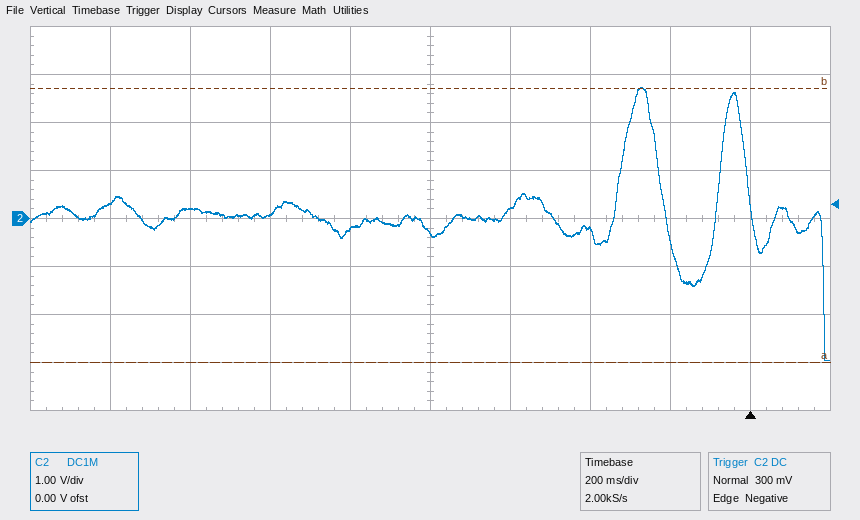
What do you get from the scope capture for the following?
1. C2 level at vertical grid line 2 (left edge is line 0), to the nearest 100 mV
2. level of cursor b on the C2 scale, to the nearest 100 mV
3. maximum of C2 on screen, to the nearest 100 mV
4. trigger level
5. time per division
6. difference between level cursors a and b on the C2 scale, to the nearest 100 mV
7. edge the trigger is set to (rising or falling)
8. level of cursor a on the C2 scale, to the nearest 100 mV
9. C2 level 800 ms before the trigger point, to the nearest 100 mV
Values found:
200 mV
2.7 V
2.7 V
300 mV
200 ms
5.7 V
falling
-3.0 V
-300 mV
